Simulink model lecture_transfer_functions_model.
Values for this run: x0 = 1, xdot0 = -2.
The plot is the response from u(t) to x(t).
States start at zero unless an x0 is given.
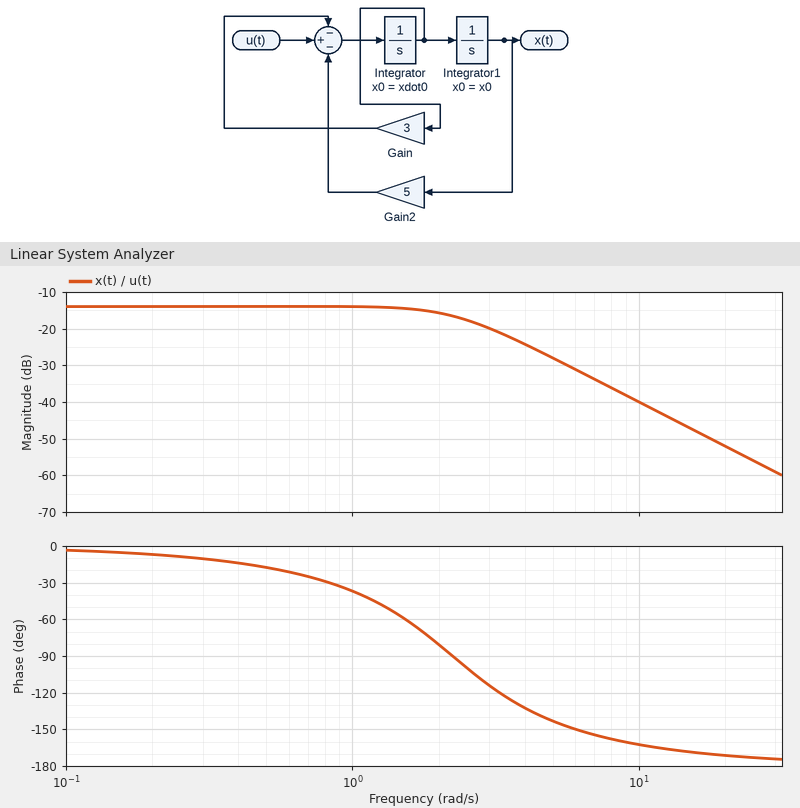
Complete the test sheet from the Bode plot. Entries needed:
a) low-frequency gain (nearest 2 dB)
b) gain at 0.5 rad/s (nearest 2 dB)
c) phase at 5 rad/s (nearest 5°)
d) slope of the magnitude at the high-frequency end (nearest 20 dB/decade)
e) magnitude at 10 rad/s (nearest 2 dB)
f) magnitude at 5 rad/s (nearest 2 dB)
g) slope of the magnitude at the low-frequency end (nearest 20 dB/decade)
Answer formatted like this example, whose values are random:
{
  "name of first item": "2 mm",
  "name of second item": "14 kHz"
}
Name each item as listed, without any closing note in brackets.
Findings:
{
  "low-frequency gain": "-14 dB",
  "gain at 0.5 rad/s": "-14 dB",
  "phase at 5 rad/s": "-145°",
  "slope of the magnitude at the high-frequency end": "-40 dB/decade",
  "magnitude at 10 rad/s": "-40 dB",
  "magnitude at 5 rad/s": "-28 dB",
  "slope of the magnitude at the low-frequency end": "0 dB/decade"
}
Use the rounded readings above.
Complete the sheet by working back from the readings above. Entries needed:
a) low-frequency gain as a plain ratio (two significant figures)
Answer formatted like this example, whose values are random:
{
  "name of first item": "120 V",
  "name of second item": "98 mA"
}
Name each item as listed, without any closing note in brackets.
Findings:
{
  "low-frequency gain as a plain ratio": "0.20"
}
